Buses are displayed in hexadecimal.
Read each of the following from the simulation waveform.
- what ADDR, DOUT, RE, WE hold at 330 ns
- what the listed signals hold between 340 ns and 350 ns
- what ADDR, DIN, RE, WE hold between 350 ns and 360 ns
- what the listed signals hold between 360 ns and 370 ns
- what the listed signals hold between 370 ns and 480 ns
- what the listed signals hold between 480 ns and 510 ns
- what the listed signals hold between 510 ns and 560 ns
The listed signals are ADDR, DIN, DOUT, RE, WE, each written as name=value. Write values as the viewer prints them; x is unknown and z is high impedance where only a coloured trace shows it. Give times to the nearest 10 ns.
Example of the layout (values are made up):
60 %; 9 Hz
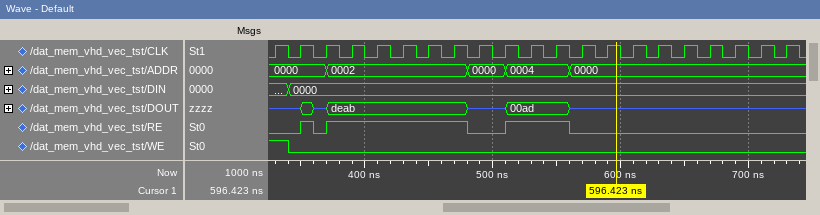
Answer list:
ADDR=0000, DOUT=z, RE=0, WE=1; ADDR=0000, DIN=0000, DOUT=z, RE=0, WE=0; ADDR=0000, DIN=0000, RE=1, WE=0; ADDR=0000, DIN=0000, DOUT=z, RE=0, WE=0; ADDR=0002, DIN=0000, DOUT=deab, RE=1, WE=0; ADDR=0000, DIN=0000, DOUT=z, RE=0, WE=0; ADDR=0004, DIN=0000, DOUT=00ad, RE=1, WE=0
